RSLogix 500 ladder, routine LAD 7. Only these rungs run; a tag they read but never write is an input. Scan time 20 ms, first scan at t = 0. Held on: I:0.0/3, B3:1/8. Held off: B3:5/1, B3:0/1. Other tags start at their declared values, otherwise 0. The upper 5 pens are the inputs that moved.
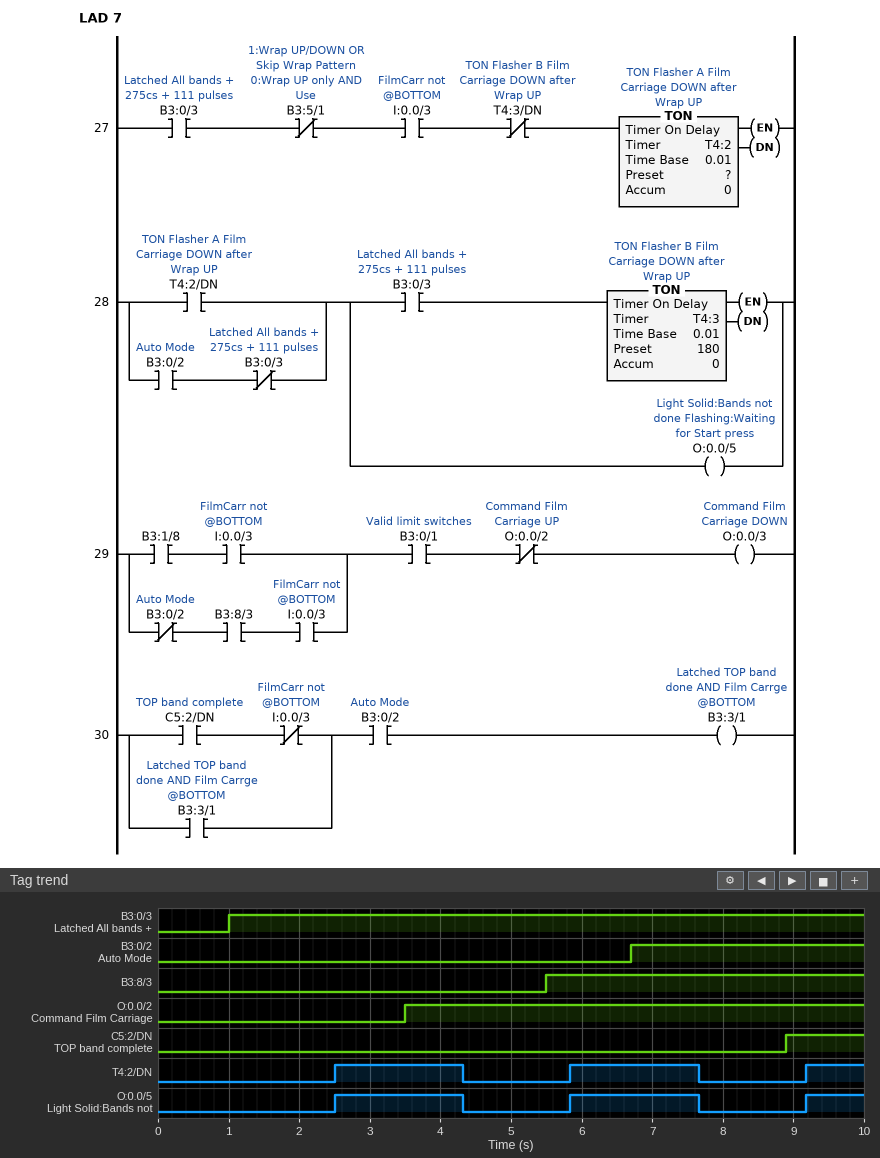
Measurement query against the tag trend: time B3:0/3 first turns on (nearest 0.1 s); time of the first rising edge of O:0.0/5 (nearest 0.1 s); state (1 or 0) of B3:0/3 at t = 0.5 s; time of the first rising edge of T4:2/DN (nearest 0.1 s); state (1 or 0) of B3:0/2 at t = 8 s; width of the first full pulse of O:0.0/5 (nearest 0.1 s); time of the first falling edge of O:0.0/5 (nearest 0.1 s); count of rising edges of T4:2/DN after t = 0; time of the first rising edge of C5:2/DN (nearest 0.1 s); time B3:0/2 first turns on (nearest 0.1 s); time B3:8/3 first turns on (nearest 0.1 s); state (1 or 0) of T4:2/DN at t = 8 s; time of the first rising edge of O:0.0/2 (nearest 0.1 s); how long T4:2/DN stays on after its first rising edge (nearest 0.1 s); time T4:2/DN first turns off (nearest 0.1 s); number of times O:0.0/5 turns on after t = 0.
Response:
1.0 s
2.5 s
0
2.5 s
1
1.8 s
4.3 s
3
8.9 s
6.7 s
5.5 s
0
3.5 s
1.8 s
4.3 s
3
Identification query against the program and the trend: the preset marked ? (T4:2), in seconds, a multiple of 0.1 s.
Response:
1.5 s
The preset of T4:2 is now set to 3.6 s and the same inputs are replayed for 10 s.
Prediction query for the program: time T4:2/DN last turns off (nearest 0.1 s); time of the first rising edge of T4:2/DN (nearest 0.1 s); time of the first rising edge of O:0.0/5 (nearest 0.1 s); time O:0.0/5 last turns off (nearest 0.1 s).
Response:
6.4 s
4.6 s
4.6 s
6.4 s
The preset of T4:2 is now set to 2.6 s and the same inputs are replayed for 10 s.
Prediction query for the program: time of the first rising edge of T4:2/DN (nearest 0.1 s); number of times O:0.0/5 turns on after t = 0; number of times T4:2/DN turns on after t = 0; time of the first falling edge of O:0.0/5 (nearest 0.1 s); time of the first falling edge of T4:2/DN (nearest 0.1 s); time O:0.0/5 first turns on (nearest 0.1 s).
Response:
3.6 s
2
2
5.4 s
5.4 s
3.6 s
